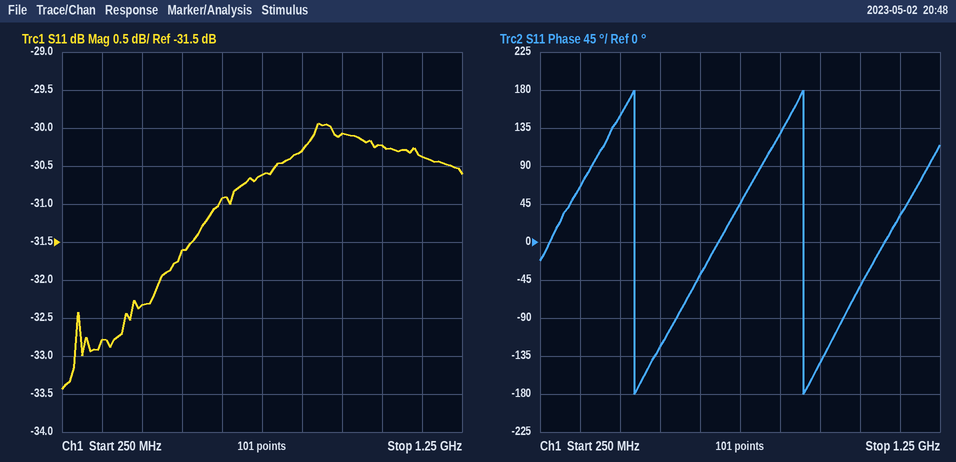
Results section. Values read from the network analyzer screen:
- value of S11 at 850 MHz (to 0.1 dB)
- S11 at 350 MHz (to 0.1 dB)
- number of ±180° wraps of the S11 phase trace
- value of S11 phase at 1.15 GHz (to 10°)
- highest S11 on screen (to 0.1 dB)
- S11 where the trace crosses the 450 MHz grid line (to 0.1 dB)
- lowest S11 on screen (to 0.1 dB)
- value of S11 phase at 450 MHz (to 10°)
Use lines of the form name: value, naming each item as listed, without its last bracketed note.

value of S11 at 850 MHz: -30.3 dB
S11 at 350 MHz: -32.8 dB
number of ±180° wraps of the S11 phase trace: 2
value of S11 phase at 1.15 GHz: 30°
highest S11 on screen: -29.9 dB
S11 where the trace crosses the 450 MHz grid line: -32.3 dB
lowest S11 on screen: -33.4 dB
value of S11 phase at 450 MHz: 150°
